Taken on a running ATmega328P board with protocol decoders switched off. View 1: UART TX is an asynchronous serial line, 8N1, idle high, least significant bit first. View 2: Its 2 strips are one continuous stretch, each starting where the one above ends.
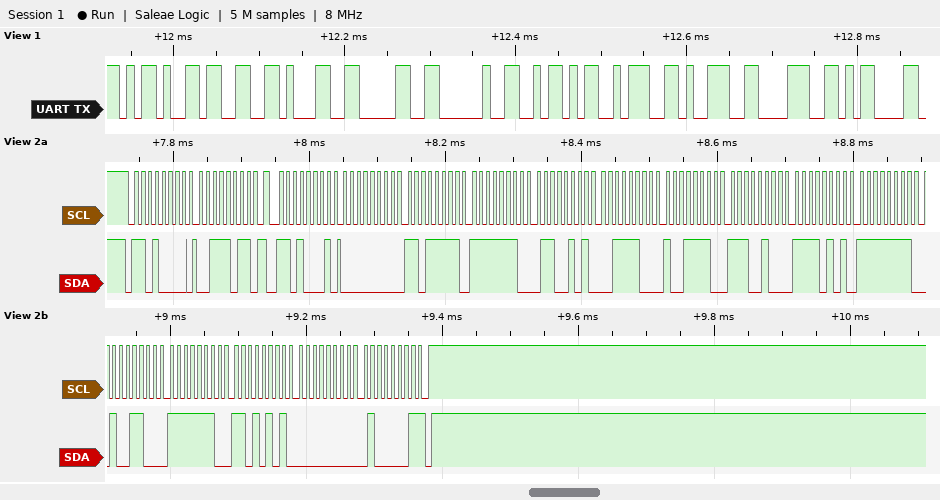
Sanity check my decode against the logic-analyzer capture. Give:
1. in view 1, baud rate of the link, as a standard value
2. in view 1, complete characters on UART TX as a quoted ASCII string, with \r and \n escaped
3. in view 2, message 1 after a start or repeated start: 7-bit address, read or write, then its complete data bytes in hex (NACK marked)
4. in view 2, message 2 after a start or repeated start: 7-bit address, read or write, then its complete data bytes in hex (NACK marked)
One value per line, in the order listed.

115200 baud
"-310 Z:98\r"
0x68 write: 3B
0x68 read: 00 DF FE 65 3C 9E E4 F5 FF 4C FE D5 00 41 NACK
